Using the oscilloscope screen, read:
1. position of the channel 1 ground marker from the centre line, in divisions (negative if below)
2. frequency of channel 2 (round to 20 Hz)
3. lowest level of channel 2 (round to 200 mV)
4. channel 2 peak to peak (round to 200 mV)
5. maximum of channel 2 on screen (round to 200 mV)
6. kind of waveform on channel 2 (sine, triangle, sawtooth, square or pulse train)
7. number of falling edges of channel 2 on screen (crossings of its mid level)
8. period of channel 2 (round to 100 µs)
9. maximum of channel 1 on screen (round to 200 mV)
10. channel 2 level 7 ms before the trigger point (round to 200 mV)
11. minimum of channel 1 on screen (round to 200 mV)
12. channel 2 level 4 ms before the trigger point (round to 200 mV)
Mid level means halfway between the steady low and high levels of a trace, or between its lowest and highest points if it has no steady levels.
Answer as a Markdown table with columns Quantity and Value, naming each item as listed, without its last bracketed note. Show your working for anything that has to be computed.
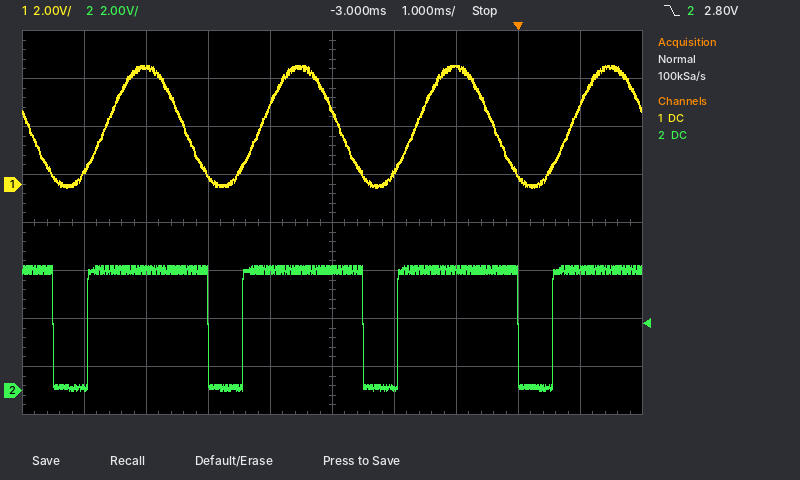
| Quantity | Value |
|---|---|
| position of the channel 1 ground marker from the centre line, in divisions | +0.8 div |
| frequency of channel 2 | 1 / 2.5 ms ≈ 400 Hz |
| lowest level of channel 2 | 0.0 V |
| channel 2 peak to peak | 5.2 V − (0.0 V) = 5.2 V |
| maximum of channel 2 on screen | 5.2 V |
| kind of waveform on channel 2 | pulse train |
| number of falling edges of channel 2 on screen | 4 |
| period of channel 2 | 2.5 ms |
| maximum of channel 1 on screen | 5.0 V |
| channel 2 level 7 ms before the trigger point | 200 mV |
| minimum of channel 1 on screen | -200 mV |
| channel 2 level 4 ms before the trigger point | 5.0 V |
